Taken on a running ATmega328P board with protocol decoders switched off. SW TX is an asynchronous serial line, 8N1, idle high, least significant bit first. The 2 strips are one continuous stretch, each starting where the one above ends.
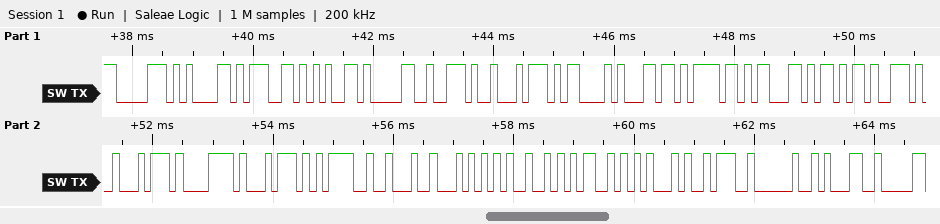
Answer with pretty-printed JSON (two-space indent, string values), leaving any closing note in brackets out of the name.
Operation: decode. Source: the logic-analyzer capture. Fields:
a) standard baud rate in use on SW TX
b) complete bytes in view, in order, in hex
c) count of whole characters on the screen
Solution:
{
  "standard baud rate in use on SW TX": "9600 baud",
  "complete bytes in view, in order, in hex": "70 61 67 65 30 2E 74 43 6C 6F 63 6B 2E 74 78 74 3D 22 54 49 4D 45 3A 20 31",
  "count of whole characters on the screen": "25"
}
